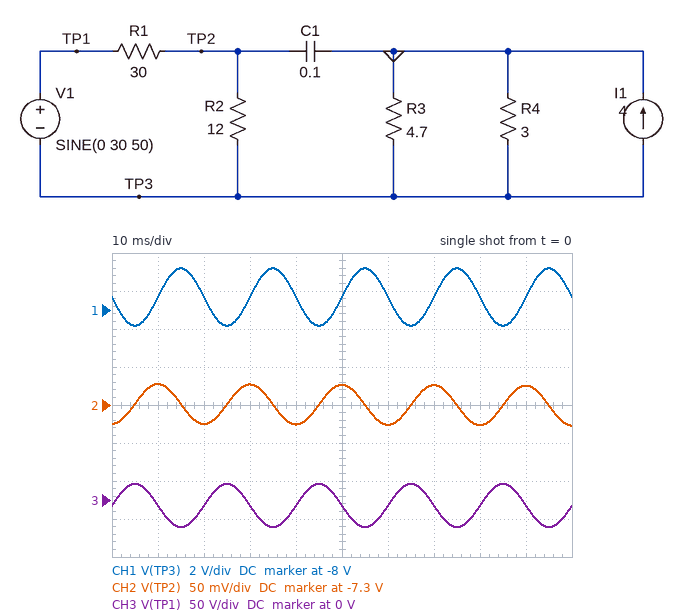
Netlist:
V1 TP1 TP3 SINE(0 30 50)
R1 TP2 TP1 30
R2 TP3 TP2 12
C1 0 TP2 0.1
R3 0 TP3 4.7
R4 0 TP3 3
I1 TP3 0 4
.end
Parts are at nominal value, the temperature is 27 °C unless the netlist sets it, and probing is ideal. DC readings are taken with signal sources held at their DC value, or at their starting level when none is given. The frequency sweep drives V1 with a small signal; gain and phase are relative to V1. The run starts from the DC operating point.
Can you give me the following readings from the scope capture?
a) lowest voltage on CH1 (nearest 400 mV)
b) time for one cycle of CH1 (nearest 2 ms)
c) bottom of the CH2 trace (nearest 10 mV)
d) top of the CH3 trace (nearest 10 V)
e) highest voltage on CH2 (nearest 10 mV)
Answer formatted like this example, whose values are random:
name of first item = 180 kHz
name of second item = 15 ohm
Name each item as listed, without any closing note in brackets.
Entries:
lowest voltage on CH1 = -8.8 V
time for one cycle of CH1 = 20 ms
bottom of the CH2 trace = -7.33 V
top of the CH3 trace = 20 V
highest voltage on CH2 = -7.27 V
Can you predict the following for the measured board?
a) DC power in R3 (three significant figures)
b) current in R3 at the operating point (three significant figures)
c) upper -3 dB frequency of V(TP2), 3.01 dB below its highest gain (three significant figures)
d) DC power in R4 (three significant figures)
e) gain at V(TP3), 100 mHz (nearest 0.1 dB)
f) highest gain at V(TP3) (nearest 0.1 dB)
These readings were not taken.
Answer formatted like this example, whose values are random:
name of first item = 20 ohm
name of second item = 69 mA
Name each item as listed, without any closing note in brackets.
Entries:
DC power in R3 = 11.4 W
current in R3 at the operating point = 1.56 A
upper -3 dB frequency of V(TP2), 3.01 dB below its highest gain = 153 mHz
DC power in R4 = 17.9 W
gain at V(TP3), 100 mHz = -31.2 dB
highest gain at V(TP3) = -26.0 dB
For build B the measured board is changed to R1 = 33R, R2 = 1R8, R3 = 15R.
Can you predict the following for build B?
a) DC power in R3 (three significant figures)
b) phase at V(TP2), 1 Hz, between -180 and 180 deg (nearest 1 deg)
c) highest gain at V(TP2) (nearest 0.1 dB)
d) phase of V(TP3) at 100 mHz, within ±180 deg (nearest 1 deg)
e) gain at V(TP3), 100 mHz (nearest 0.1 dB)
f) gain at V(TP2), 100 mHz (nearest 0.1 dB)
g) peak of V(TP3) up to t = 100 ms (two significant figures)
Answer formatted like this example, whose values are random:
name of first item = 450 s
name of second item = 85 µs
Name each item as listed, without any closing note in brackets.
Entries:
DC power in R3 = 6.67 W
phase at V(TP2), 1 Hz, between -180 and 180 deg = -69 deg
highest gain at V(TP2) = -25.7 dB
phase of V(TP3) at 100 mHz, within ±180 deg = -105 deg
gain at V(TP3), 100 mHz = -42.1 dB
gain at V(TP2), 100 mHz = -26.0 dB
peak of V(TP3) up to t = 100 ms = -9.1 V
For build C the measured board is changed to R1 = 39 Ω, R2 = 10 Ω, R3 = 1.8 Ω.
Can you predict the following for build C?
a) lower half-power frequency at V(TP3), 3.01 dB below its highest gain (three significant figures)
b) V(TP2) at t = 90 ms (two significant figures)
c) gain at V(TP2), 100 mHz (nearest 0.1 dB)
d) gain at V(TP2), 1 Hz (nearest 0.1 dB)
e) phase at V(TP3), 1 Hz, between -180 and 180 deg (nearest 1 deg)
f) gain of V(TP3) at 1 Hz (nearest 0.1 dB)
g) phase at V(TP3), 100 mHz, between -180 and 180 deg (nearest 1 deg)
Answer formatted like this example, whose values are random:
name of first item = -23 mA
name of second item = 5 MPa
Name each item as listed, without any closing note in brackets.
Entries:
lower half-power frequency at V(TP3), 3.01 dB below its highest gain = 175 mHz
V(TP2) at t = 90 ms = -4.5 V
gain at V(TP2), 100 mHz = -15.0 dB
gain at V(TP2), 1 Hz = -29.1 dB
phase at V(TP3), 1 Hz, between -180 and 180 deg = -170 deg
gain of V(TP3) at 1 Hz = -32.1 dB
phase at V(TP3), 100 mHz, between -180 and 180 deg = -120 deg
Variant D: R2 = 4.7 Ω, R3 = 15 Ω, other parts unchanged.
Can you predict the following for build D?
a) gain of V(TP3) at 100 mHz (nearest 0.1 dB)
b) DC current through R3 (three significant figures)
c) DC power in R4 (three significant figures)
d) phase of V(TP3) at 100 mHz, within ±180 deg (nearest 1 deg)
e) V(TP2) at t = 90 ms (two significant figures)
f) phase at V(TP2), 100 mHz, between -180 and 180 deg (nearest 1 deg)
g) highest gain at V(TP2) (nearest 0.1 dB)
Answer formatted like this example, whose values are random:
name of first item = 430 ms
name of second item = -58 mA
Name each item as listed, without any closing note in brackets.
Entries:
gain of V(TP3) at 100 mHz = -34.1 dB
DC current through R3 = 667 mA
DC power in R4 = 33.3 W
phase of V(TP3) at 100 mHz, within ±180 deg = -112 deg
V(TP2) at t = 90 ms = -10 V
phase at V(TP2), 100 mHz, between -180 and 180 deg = -22 deg
highest gain at V(TP2) = -17.4 dB
